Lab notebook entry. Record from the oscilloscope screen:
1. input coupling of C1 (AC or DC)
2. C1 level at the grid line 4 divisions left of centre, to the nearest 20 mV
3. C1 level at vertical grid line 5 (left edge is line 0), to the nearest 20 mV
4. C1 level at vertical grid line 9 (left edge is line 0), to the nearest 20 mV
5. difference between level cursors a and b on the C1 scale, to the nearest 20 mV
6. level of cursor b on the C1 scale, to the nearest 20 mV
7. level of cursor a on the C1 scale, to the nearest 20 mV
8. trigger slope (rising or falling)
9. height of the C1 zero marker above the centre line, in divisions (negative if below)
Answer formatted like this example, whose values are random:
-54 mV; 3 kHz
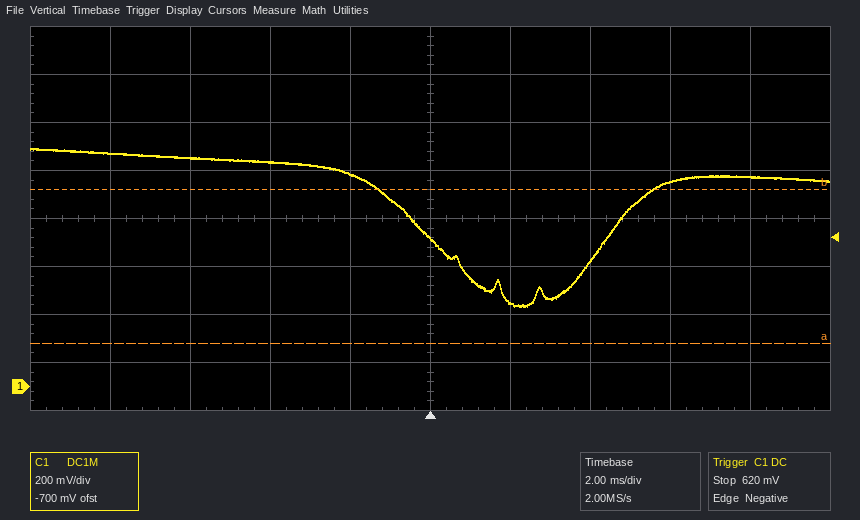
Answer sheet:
DC; 980 mV; 620 mV; 880 mV; 640 mV; 820 mV; 180 mV; falling; -3.5 div
